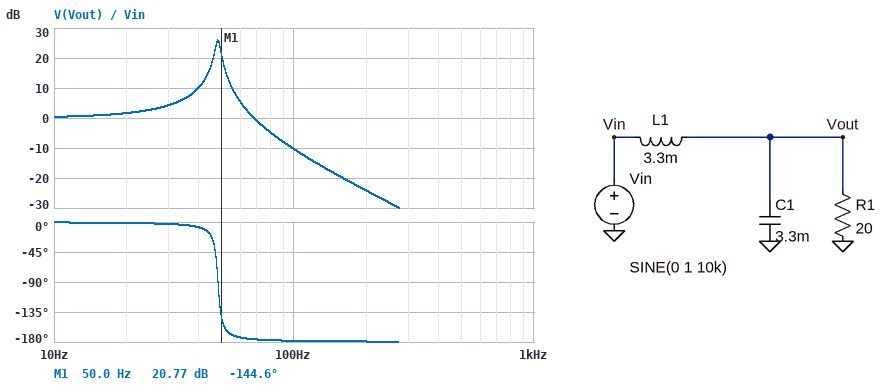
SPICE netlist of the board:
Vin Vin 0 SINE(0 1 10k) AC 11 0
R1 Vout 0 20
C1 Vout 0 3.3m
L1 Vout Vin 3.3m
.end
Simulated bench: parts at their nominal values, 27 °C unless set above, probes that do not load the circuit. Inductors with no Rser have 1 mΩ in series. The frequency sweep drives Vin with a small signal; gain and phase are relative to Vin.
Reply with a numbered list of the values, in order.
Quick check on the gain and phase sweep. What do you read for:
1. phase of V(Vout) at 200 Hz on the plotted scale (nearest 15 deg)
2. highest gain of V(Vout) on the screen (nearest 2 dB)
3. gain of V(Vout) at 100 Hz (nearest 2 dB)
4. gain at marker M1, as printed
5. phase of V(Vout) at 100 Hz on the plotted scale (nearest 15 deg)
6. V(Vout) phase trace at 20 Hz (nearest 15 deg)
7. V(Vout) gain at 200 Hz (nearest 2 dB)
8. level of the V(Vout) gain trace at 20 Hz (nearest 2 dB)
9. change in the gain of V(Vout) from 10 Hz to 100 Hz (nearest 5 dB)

1. -180 deg
2. 26 dB
3. -10 dB
4. 20.77 dB
5. -180 deg
6. 0 deg
7. -24 dB
8. 2 dB
9. -10 dB
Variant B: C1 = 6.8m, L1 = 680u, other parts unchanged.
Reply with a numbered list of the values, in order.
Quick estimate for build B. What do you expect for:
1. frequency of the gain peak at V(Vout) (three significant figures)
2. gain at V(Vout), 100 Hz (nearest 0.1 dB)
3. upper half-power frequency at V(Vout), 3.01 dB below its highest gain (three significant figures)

1. 74.0 Hz
2. 1.7 dB
3. 74.7 Hz
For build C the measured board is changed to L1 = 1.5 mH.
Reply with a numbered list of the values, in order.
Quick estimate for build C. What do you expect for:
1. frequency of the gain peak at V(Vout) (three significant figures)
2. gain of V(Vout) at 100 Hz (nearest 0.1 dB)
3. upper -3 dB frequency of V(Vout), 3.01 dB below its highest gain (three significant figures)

1. 71.5 Hz
2. 0.4 dB
3. 72.8 Hz
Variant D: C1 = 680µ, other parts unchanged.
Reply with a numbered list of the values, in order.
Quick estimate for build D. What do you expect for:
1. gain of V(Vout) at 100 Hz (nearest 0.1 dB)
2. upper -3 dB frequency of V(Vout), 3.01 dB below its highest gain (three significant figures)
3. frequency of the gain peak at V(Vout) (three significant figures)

1. 16.2 dB
2. 112 Hz
3. 106 Hz
